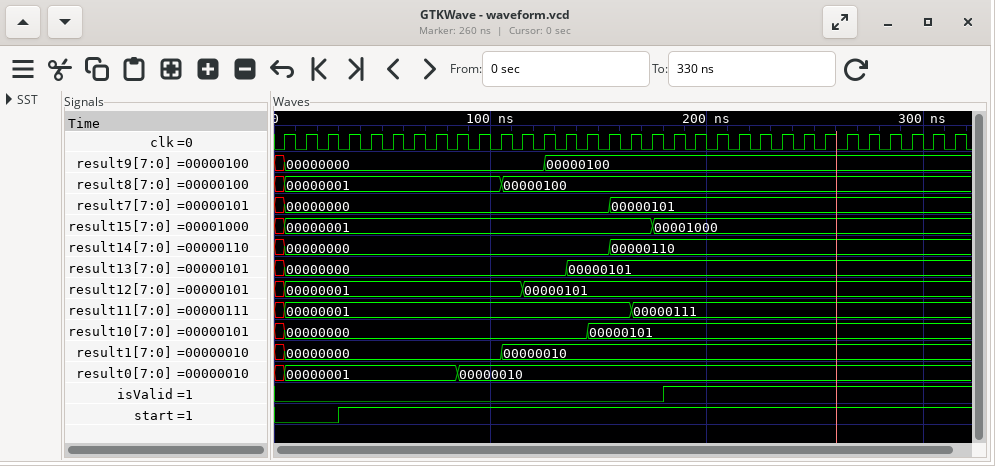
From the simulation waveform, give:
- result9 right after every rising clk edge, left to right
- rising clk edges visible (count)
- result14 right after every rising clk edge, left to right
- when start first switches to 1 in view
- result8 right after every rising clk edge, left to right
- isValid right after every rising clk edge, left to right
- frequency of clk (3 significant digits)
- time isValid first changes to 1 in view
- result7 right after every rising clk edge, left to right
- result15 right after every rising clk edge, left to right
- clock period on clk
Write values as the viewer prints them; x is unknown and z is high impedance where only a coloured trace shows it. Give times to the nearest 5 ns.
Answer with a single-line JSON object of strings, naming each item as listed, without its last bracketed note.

{"result9 right after every rising clk edge, left to right": "00000000, 00000000, 00000000, 00000000, 00000000, 00000000, 00000000, 00000000, 00000000, 00000000, 00000000, 00000000, 00000100, 00000100, 00000100, 00000100, 00000100, 00000100, 00000100, 00000100, 00000100, 00000100, 00000100, 00000100, 00000100, 00000100, 00000100, 00000100, 00000100, 00000100, 00000100, 00000100", "rising clk edges visible": "32", "result14 right after every rising clk edge, left to right": "00000000, 00000000, 00000000, 00000000, 00000000, 00000000, 00000000, 00000000, 00000000, 00000000, 00000000, 00000000, 00000000, 00000000, 00000000, 00000110, 00000110, 00000110, 00000110, 00000110, 00000110, 00000110, 00000110, 00000110, 00000110, 00000110, 00000110, 00000110, 00000110, 00000110, 00000110, 00000110", "when start first switches to 1 in view": "30 ns", "result8 right after every rising clk edge, left to right": "00000001, 00000001, 00000001, 00000001, 00000001, 00000001, 00000001, 00000001, 00000001, 00000001, 00000100, 00000100, 00000100, 00000100, 00000100, 00000100, 00000100, 00000100, 00000100, 00000100, 00000100, 00000100, 00000100, 00000100, 00000100, 00000100, 00000100, 00000100, 00000100, 00000100, 00000100, 00000100", "isValid right after every rising clk edge, left to right": "0 0 0 0 0 0 0 0 0 0 0 0 0 0 0 0 0 0 1 1 1 1 1 1 1 1 1 1 1 1 1 1", "frequency of clk": "100 MHz", "time isValid first changes to 1 in view": "180 ns", "result7 right after every rising clk edge, left to right": "00000000, 00000000, 00000000, 00000000, 00000000, 00000000, 00000000, 00000000, 00000000, 00000000, 00000000, 00000000, 00000000, 00000000, 00000000, 00000101, 00000101, 00000101, 00000101, 00000101, 00000101, 00000101, 00000101, 00000101, 00000101, 00000101, 00000101, 00000101, 00000101, 00000101, 00000101, 00000101", "result15 right after every rising clk edge, left to right": "00000001, 00000001, 00000001, 00000001, 00000001, 00000001, 00000001, 00000001, 00000001, 00000001, 00000001, 00000001, 00000001, 00000001, 00000001, 00000001, 00000001, 00001000, 00001000, 00001000, 00001000, 00001000, 00001000, 00001000, 00001000, 00001000, 00001000, 00001000, 00001000, 00001000, 00001000, 00001000", "clock period on clk": "10 ns"}
